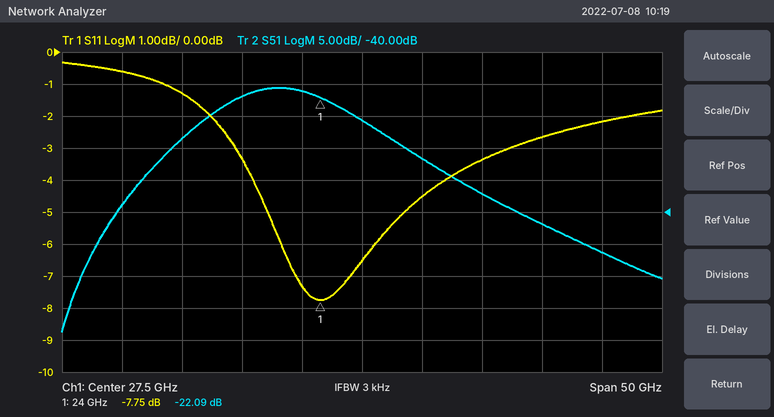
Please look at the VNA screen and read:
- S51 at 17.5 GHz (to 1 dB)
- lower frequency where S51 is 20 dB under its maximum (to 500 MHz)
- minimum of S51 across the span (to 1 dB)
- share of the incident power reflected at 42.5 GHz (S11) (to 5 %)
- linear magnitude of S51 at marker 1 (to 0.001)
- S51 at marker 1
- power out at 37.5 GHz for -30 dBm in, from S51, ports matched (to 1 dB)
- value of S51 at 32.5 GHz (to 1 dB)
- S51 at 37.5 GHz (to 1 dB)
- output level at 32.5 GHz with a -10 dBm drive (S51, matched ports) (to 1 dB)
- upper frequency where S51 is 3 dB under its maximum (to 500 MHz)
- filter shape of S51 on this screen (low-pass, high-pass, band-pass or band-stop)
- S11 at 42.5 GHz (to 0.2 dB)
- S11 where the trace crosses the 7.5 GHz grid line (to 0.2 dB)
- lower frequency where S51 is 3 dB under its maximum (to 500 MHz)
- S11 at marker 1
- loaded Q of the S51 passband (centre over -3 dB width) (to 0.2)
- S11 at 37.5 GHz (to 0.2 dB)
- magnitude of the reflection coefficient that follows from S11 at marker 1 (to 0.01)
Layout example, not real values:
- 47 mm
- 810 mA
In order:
- -22 dB
- 7.0 GHz
- -59 dB
- 55 %
- 0.079
- -22.09 dB
- -67 dBm
- -32 dB
- -37 dB
- -42 dBm
- 25.5 GHz
- band-pass
- -2.6 dB
- -0.6 dB
- 16.0 GHz
- -7.75 dB
- 2.2
- -3.4 dB
- 0.41
